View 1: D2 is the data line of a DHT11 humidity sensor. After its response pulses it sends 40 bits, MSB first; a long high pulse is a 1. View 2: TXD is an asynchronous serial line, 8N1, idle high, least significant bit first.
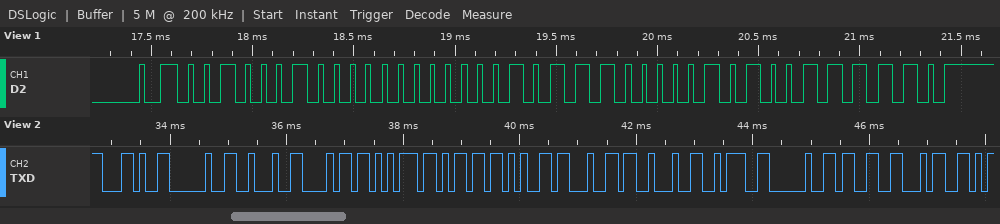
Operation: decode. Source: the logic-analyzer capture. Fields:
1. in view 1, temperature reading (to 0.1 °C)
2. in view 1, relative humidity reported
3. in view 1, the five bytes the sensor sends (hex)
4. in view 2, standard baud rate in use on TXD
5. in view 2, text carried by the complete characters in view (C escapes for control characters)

23.5 °C
34 %
22 00 17 05 3E
9600 baud
", \"humed\": 34"
